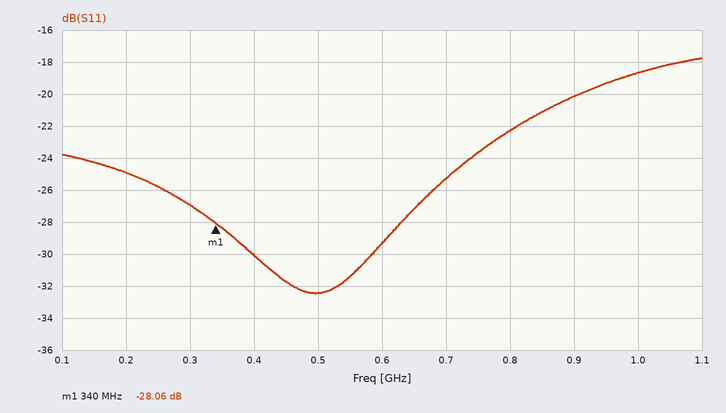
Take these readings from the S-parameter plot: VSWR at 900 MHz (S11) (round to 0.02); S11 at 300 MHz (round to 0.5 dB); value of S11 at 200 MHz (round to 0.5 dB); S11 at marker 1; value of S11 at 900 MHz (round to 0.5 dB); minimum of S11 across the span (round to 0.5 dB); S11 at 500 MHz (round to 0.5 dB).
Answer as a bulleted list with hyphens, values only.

- 1.22
- -27.0 dB
- -25.0 dB
- -28.06 dB
- -20.0 dB
- -32.5 dB
- -32.5 dB
